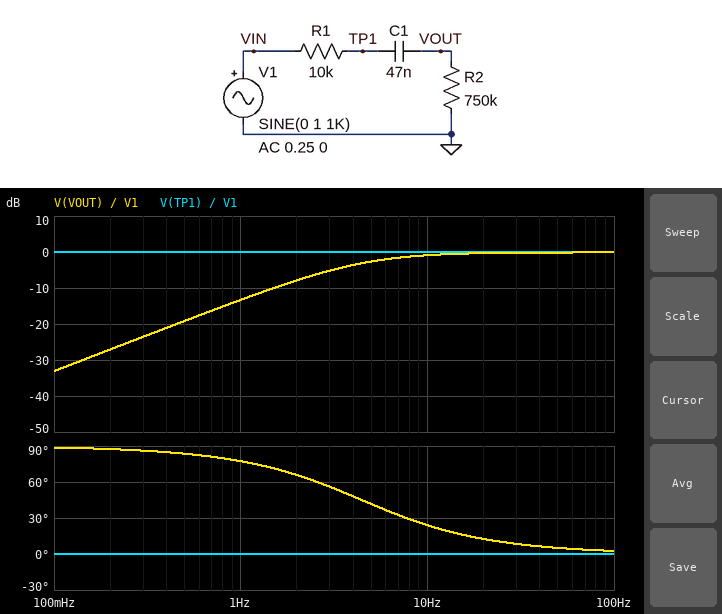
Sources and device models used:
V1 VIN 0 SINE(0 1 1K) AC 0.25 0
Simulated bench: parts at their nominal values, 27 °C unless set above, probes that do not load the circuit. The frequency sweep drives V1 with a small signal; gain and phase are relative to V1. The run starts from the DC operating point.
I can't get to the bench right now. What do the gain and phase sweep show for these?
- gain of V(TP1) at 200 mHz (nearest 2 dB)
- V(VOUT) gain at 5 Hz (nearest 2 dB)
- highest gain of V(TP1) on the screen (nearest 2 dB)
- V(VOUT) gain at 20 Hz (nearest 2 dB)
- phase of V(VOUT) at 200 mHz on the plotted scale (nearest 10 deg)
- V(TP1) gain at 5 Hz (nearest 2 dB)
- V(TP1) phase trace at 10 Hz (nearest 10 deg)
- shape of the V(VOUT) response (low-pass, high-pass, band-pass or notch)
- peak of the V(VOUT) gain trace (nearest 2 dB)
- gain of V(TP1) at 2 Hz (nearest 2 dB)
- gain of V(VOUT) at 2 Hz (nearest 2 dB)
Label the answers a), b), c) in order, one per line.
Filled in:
a) 0 dB
b) -2 dB
c) 0 dB
d) 0 dB
e) 90 deg
f) 0 dB
g) 0 deg
h) high-pass
i) 0 dB
j) 0 dB
k) -8 dB
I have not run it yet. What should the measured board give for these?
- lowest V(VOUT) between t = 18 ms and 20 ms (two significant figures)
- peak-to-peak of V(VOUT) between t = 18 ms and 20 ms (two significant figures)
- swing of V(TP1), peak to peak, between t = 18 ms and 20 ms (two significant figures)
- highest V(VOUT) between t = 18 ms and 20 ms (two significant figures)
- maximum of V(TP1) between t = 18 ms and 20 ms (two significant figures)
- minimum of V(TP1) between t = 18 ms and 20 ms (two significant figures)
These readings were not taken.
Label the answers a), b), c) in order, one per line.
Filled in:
a) -990 mV
b) 2.0 V
c) 2.0 V
d) 980 mV
e) 990 mV
f) -990 mV
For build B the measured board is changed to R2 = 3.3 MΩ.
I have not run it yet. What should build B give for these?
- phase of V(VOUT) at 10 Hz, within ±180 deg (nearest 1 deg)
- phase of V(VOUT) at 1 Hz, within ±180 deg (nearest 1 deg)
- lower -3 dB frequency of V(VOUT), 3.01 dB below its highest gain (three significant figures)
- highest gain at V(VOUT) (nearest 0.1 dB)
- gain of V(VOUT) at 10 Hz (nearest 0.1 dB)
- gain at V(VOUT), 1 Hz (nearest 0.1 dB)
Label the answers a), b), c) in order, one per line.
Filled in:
a) 6 deg
b) 46 deg
c) 1.02 Hz
d) 0 dB
e) -0.1 dB
f) -3.1 dB
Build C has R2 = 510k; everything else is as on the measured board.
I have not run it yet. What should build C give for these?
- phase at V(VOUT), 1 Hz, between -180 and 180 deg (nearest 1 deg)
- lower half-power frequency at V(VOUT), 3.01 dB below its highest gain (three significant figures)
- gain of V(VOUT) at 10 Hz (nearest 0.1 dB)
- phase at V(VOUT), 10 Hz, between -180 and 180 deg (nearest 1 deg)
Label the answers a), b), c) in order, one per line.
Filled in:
a) 81 deg
b) 6.51 Hz
c) -1.7 dB
d) 33 deg
